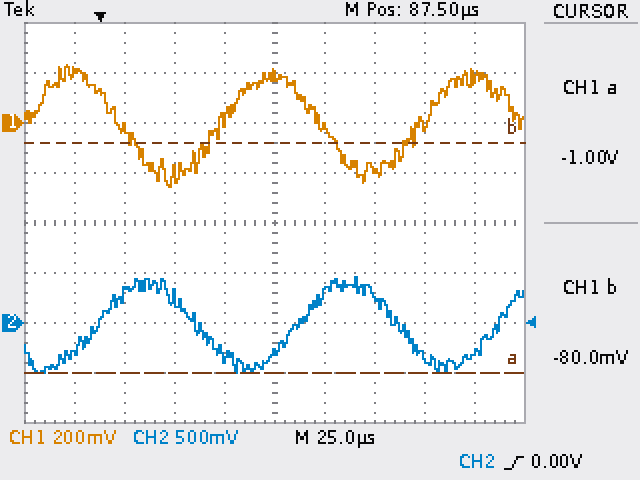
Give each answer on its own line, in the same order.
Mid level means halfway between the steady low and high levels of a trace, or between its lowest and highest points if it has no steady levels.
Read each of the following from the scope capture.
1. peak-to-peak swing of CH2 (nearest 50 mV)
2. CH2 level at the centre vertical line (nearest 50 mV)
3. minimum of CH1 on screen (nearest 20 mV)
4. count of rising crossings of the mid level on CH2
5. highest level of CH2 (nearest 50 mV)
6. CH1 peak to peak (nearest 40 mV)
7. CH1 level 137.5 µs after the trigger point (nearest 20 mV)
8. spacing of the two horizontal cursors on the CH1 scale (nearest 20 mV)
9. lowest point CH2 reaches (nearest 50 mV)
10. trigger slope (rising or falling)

950 mV
-300 mV
-260 mV
3
450 mV
480 mV
-180 mV
920 mV
-500 mV
rising
